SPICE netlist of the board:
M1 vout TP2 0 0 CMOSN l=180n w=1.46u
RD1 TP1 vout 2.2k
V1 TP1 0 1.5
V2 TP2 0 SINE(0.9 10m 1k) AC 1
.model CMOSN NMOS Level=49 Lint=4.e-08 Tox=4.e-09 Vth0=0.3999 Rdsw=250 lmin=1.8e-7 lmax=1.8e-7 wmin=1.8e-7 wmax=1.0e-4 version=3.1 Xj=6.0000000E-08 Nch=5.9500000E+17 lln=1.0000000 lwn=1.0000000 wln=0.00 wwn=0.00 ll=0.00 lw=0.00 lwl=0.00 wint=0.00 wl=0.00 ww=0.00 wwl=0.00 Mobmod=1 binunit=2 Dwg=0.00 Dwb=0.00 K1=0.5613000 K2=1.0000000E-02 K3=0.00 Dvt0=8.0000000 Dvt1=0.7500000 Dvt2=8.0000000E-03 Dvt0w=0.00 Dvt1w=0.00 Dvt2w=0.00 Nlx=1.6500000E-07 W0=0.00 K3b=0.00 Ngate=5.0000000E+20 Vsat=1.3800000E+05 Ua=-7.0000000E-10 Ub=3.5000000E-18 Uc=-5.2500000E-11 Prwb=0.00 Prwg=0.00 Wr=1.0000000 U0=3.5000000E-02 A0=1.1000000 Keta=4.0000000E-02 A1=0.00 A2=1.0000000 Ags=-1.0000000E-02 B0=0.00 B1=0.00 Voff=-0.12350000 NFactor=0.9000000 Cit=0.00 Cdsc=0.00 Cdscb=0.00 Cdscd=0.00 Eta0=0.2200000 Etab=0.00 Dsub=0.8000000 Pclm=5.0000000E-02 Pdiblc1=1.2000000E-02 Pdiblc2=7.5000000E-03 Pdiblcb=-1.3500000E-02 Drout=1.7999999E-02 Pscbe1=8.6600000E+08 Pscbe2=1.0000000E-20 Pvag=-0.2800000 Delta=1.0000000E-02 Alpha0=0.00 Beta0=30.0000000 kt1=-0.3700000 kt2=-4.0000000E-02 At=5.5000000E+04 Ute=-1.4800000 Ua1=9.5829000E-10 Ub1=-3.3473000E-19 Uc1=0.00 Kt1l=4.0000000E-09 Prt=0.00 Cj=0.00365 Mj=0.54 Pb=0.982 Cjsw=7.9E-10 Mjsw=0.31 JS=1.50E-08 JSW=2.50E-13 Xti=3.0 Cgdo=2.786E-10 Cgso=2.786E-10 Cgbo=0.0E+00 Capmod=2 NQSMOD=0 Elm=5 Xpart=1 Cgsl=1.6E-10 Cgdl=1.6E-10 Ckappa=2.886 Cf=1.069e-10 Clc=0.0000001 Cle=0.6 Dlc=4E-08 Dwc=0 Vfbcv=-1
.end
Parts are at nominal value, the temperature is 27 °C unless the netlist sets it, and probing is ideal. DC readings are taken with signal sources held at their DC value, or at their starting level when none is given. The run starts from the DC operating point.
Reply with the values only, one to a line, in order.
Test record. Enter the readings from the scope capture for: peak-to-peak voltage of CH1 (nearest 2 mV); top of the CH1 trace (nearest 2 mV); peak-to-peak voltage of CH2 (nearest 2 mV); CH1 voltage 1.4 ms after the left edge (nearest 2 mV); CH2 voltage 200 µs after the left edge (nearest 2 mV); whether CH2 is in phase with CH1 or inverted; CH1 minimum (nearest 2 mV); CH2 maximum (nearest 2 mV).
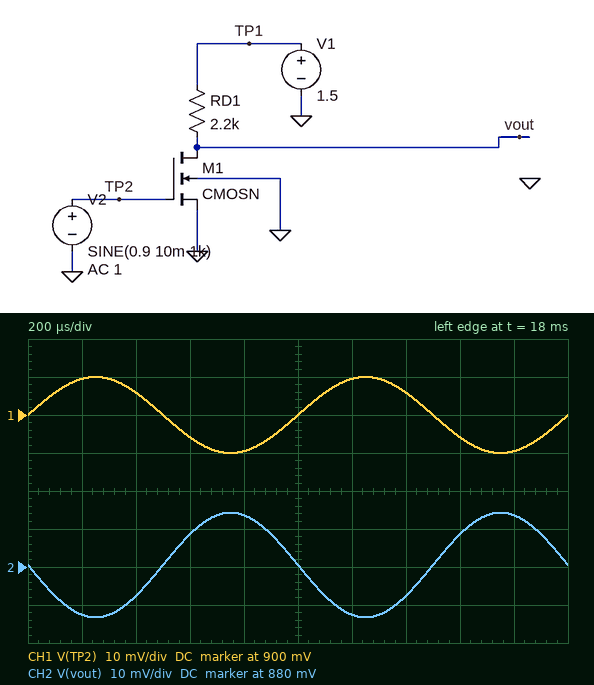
20 mV
910 mV
28 mV
906 mV
868 mV
inverted
890 mV
894 mV
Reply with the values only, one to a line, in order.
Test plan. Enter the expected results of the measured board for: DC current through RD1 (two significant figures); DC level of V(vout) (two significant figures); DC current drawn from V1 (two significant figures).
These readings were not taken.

280 µA
880 mV
280 µA
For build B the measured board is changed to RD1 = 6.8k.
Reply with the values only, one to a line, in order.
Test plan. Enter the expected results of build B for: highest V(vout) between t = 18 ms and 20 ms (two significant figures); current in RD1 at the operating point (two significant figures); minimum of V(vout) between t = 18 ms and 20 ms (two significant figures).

220 mV
190 µA
210 mV
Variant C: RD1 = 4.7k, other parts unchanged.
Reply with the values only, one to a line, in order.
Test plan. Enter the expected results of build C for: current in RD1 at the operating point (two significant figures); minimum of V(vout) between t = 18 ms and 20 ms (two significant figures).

240 µA
370 mV
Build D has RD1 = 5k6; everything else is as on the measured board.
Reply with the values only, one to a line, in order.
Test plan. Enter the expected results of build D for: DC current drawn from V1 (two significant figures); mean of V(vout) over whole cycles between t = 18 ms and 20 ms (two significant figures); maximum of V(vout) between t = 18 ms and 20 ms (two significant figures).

220 µA
290 mV
300 mV
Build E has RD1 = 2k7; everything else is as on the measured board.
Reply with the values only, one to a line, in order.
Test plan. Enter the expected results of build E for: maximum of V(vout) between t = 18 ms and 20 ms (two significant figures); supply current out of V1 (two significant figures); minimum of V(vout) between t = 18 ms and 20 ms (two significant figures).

780 mV
270 µA
750 mV
